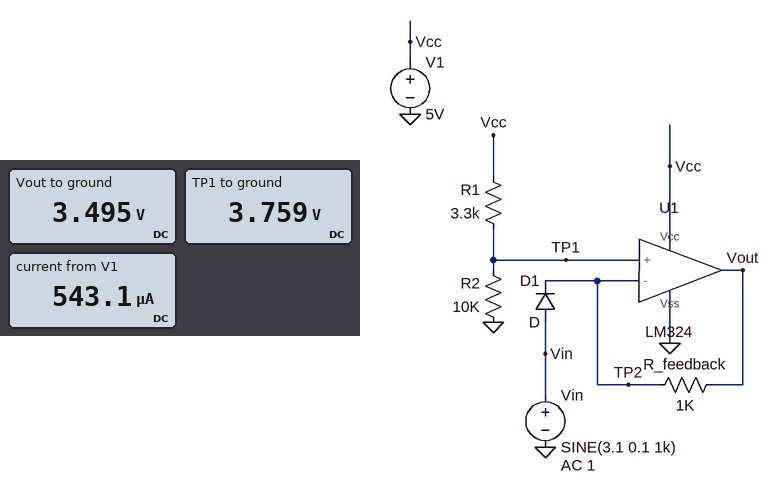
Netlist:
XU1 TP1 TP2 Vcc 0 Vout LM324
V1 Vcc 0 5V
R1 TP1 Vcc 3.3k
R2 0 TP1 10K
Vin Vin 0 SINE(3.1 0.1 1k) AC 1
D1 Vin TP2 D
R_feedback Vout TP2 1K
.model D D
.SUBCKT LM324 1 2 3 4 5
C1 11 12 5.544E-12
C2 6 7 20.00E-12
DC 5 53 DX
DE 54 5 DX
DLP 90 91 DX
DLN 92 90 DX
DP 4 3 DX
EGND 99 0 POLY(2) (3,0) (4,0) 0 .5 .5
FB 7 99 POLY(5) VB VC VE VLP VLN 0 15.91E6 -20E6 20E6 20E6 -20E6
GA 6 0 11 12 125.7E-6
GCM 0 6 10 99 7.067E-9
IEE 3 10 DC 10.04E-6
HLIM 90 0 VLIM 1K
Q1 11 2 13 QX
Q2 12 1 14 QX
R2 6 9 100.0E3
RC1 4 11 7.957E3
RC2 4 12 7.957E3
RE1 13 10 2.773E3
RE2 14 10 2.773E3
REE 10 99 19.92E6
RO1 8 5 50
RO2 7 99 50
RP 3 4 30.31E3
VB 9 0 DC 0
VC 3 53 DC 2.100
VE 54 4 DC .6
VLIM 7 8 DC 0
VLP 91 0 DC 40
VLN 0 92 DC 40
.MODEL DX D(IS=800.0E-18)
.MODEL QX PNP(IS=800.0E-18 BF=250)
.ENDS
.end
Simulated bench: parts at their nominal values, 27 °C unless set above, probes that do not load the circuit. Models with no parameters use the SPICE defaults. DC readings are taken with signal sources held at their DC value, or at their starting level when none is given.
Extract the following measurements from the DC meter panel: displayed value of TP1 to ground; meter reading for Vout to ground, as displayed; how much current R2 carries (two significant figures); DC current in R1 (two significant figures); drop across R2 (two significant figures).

3.759 V
3.495 V
380 µA
380 µA
3.8 V
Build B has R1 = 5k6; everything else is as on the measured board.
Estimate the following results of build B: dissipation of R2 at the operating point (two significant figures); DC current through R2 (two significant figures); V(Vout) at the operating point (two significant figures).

1.0 mW
320 µA
3.2 V
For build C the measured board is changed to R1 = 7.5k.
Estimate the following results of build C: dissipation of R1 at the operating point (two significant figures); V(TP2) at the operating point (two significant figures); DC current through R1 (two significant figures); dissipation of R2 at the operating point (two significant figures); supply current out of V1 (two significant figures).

610 µW
2.9 V
290 µA
820 µW
460 µA
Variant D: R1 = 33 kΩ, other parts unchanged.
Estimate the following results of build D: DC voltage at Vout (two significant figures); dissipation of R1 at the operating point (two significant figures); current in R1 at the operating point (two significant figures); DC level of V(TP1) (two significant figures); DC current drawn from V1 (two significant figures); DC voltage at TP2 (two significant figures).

4.5 mV
450 µW
120 µA
1.2 V
290 µA
2.4 V
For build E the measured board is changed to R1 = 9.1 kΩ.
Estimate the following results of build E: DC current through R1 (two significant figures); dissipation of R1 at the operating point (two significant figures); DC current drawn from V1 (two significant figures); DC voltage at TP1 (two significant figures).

260 µA
620 µW
440 µA
2.6 V
